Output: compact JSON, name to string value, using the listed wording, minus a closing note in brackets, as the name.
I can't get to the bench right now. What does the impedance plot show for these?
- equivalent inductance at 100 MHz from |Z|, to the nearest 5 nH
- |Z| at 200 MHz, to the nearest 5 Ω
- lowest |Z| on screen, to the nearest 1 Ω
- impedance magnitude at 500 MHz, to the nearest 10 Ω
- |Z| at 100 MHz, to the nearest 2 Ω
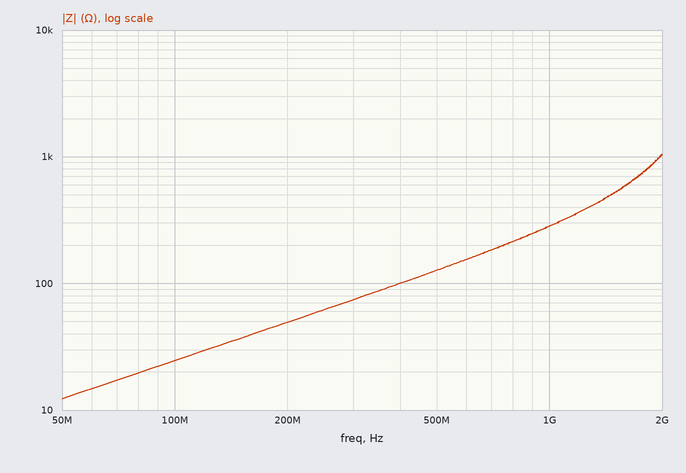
{"equivalent inductance at 100 MHz from |Z|, to the nearest 5 nH": "40 nH", "|Z| at 200 MHz, to the nearest 5 Ω": "50 Ω", "lowest |Z| on screen, to the nearest 1 Ω": "12 Ω", "impedance magnitude at 500 MHz, to the nearest 10 Ω": "130 Ω", "|Z| at 100 MHz, to the nearest 2 Ω": "24 Ω"}
